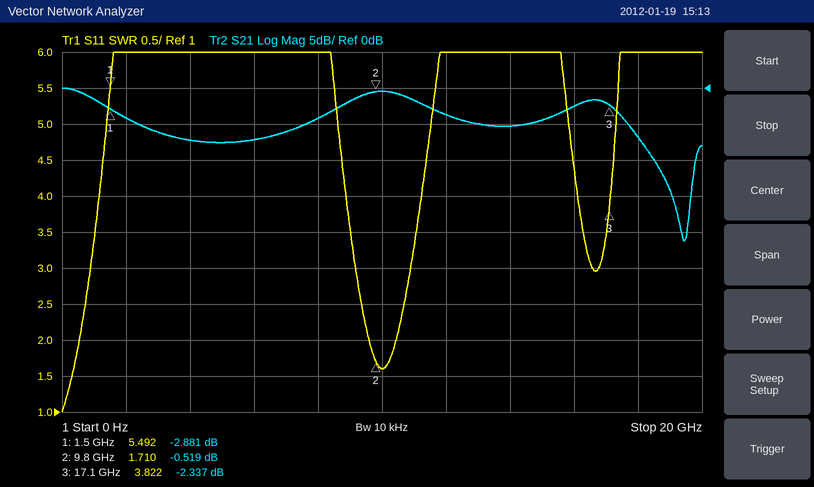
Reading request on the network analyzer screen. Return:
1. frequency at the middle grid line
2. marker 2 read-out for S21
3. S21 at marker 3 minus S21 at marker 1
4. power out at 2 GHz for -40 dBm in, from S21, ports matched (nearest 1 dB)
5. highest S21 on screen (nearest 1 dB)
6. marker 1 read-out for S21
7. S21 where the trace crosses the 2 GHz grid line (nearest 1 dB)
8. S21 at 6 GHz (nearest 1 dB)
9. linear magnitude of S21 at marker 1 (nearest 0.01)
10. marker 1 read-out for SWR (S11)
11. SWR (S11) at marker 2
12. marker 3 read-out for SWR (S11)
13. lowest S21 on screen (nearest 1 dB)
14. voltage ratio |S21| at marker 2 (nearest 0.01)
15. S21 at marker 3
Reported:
10 GHz
-0.519 dB
0.544 dB
-44 dBm
0 dB
-2.881 dB
-4 dB
-7 dB
0.72
5.492
1.710
3.822
-21 dB
0.94
-2.337 dB
